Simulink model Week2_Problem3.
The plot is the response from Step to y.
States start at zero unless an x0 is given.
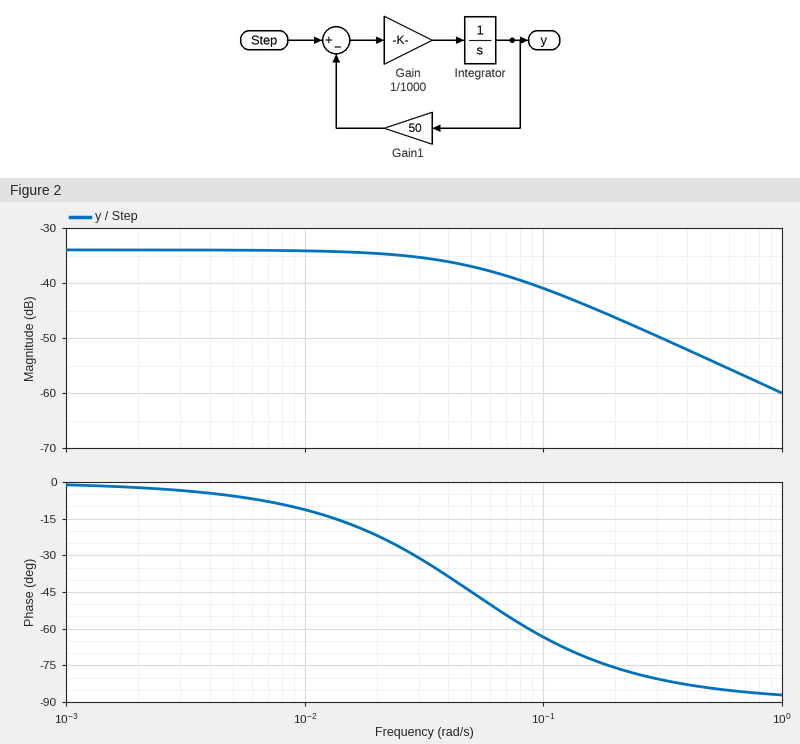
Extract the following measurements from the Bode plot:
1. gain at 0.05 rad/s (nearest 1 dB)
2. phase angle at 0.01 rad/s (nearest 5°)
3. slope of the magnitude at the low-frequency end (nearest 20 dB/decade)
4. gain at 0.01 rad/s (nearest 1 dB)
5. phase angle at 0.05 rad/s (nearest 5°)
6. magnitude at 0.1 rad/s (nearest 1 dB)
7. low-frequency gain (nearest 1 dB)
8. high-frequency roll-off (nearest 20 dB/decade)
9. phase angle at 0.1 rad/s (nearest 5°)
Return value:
-37 dB
-10°
0 dB/decade
-34 dB
-45°
-41 dB
-34 dB
-20 dB/decade
-65°
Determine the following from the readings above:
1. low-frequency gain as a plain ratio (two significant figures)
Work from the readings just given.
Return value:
0.020
